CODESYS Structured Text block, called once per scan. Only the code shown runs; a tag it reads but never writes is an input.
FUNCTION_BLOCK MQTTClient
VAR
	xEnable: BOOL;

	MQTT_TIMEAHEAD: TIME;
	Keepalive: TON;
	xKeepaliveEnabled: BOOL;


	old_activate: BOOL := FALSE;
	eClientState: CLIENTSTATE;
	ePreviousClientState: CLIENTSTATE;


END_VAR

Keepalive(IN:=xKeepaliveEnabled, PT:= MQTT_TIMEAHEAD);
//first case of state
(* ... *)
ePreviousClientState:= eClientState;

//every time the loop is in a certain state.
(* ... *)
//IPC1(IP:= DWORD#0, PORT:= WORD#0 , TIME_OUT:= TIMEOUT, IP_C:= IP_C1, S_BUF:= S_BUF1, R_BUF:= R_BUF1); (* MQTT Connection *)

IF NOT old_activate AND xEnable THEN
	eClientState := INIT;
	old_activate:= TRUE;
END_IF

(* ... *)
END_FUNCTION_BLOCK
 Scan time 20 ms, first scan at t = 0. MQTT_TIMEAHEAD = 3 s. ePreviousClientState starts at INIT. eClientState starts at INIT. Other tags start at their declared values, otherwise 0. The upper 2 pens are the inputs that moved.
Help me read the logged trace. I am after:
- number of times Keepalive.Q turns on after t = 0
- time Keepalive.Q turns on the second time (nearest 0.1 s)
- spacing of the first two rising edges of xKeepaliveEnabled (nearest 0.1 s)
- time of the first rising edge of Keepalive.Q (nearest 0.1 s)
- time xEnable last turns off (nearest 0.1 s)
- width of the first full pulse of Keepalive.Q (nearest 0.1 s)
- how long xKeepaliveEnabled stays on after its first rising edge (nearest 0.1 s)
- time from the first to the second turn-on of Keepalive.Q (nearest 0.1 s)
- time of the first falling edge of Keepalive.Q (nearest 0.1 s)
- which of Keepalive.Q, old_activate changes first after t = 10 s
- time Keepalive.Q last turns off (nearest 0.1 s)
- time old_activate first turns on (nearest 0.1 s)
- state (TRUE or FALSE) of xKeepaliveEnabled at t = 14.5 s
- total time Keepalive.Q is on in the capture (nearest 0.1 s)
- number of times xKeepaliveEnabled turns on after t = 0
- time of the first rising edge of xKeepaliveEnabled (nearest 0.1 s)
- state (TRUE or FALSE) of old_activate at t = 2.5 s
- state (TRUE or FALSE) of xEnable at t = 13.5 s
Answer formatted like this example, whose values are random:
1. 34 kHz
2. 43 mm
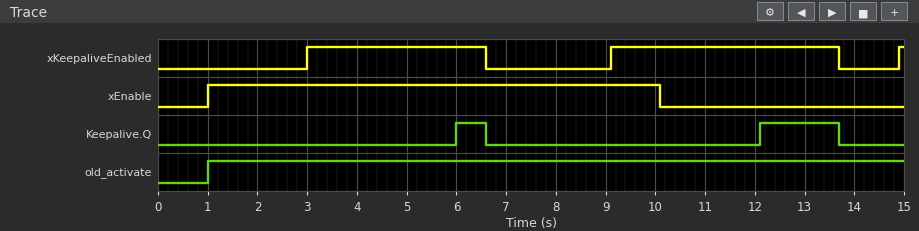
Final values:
1. 2
2. 12.1 s
3. 6.1 s
4. 6.0 s
5. 10.1 s
6. 0.6 s
7. 3.6 s
8. 6.1 s
9. 6.6 s
10. Keepalive.Q
11. 13.7 s
12. 1.0 s
13. FALSE
14. 2.2 s
15. 3
16. 3.0 s
17. TRUE
18. FALSE
